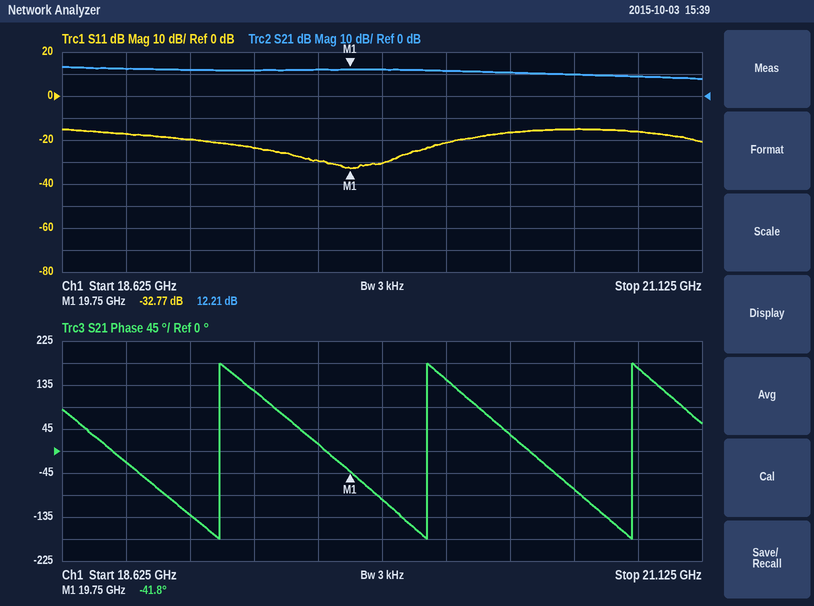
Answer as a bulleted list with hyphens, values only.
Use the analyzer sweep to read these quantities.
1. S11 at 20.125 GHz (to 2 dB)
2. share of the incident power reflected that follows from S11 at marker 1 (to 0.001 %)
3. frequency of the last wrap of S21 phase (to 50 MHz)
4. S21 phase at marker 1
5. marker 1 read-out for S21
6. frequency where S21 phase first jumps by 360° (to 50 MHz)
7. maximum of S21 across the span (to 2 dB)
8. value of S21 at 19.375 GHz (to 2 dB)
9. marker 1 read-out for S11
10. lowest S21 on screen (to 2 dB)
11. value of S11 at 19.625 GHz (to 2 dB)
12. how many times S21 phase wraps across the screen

- -22 dB
- 0.053 %
- 20.85 GHz
- -41.8°
- 12.21 dB
- 19.25 GHz
- 14 dB
- 12 dB
- -32.77 dB
- 8 dB
- -30 dB
- 3
